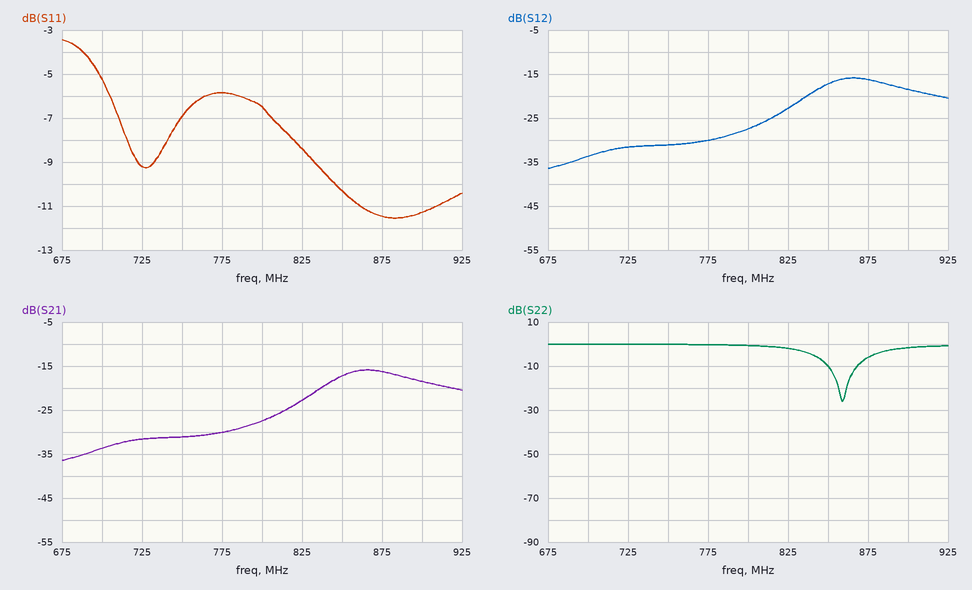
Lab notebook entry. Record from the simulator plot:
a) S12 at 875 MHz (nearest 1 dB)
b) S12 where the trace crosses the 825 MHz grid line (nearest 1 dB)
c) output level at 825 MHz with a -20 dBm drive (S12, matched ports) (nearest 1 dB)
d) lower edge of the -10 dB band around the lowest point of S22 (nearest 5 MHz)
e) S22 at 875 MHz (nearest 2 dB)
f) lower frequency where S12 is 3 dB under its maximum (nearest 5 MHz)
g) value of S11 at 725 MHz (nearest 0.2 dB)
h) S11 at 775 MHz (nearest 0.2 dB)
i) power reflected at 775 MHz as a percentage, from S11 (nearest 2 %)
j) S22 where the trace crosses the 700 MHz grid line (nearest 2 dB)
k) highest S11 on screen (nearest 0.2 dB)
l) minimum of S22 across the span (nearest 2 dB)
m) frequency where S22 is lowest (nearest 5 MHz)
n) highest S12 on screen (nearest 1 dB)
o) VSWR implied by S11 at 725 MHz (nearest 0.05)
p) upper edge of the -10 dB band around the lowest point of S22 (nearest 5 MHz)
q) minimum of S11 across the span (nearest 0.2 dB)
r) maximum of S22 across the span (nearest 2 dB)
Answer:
-16 dB
-23 dB
-43 dBm
850 MHz
-6 dB
840 MHz
-9.2 dB
-5.8 dB
26 %
0 dB
-3.4 dB
-26 dB
860 MHz
-16 dB
2.05
870 MHz
-11.6 dB
0 dB
